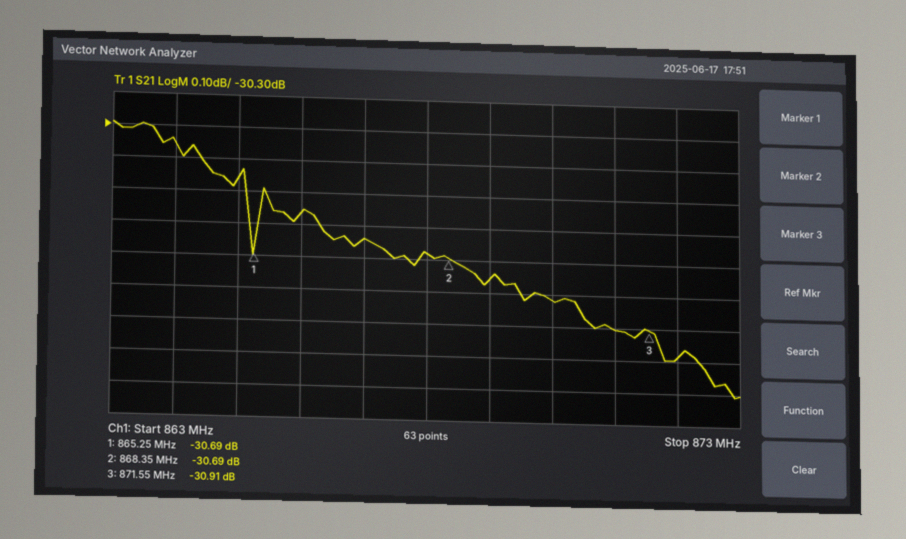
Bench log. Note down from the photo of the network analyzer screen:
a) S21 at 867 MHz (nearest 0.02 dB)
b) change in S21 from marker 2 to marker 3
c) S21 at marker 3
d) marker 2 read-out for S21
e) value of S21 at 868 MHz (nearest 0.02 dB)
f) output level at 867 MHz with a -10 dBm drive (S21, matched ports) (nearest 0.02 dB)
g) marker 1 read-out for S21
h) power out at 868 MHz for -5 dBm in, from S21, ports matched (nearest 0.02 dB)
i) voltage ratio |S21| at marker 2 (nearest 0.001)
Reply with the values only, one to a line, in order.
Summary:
-30.64 dB
-0.22 dB
-30.91 dB
-30.69 dB
-30.68 dB
-40.64 dBm
-30.69 dB
-35.68 dBm
0.029
